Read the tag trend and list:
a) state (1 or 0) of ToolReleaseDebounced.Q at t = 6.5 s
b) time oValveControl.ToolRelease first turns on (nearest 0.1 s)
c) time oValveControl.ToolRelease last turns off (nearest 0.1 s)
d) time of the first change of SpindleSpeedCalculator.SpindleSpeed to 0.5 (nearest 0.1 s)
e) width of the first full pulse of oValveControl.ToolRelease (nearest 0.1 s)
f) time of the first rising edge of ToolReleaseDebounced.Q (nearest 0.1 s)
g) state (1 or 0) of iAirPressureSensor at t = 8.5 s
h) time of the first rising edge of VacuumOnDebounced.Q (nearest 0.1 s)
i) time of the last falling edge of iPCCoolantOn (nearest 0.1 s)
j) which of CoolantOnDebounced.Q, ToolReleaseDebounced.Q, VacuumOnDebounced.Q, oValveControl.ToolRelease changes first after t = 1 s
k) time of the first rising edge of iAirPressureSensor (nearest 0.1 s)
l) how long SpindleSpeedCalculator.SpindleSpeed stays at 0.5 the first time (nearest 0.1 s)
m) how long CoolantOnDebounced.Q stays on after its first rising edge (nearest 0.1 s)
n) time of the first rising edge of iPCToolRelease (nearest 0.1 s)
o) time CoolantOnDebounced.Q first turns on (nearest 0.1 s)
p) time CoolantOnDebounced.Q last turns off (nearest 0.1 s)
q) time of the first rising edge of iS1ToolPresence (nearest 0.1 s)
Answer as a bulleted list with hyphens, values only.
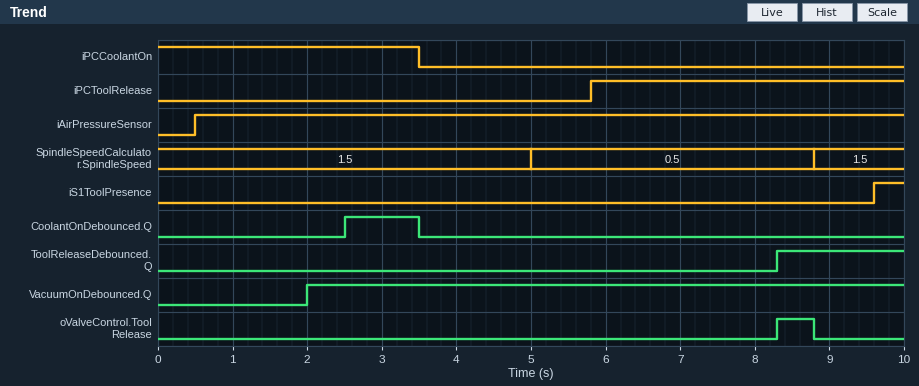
- 0
- 8.3 s
- 8.8 s
- 5.0 s
- 0.5 s
- 8.3 s
- 1
- 2.0 s
- 3.5 s
- VacuumOnDebounced.Q
- 0.5 s
- 3.8 s
- 1.0 s
- 5.8 s
- 2.5 s
- 3.5 s
- 9.6 s
